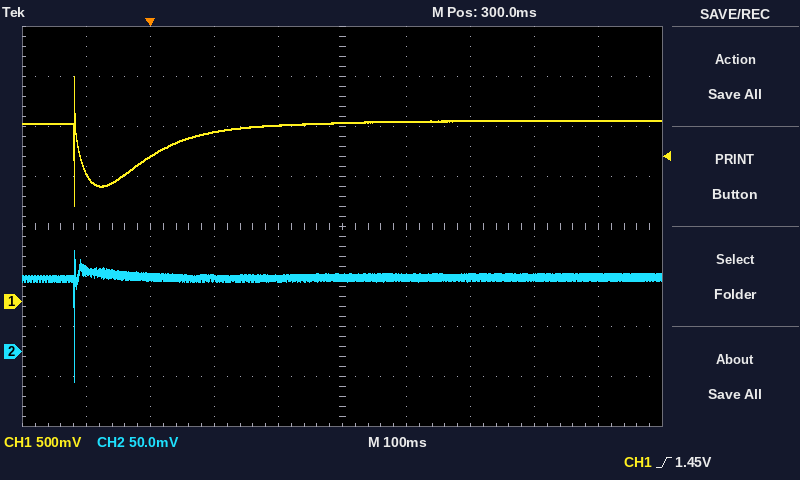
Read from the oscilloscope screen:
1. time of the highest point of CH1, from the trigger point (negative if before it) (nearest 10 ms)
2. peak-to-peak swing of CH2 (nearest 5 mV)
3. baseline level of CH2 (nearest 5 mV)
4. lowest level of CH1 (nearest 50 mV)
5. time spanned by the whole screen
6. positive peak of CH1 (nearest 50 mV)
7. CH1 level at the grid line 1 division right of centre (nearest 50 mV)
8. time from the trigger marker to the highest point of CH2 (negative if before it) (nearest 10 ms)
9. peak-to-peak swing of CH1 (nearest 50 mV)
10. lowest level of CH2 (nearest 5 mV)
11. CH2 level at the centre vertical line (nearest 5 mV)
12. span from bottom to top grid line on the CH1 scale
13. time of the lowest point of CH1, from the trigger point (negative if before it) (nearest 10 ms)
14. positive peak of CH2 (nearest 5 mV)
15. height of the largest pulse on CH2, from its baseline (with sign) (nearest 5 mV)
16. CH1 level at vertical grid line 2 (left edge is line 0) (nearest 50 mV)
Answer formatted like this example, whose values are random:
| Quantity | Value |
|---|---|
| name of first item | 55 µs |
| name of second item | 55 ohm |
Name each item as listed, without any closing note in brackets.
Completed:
| Quantity | Value |
|---|---|
| time of the highest point of CH1, from the trigger point (negative if before it) | -120 ms |
| peak-to-peak swing of CH2 | 130 mV |
| baseline level of CH2 | 75 mV |
| lowest level of CH1 | 950 mV |
| time spanned by the whole screen | 1 s |
| positive peak of CH1 | 2.25 V |
| CH1 level at the grid line 1 division right of centre | 1.80 V |
| time from the trigger marker to the highest point of CH2 (negative if before it) | -120 ms |
| peak-to-peak swing of CH1 | 1.30 V |
| lowest level of CH2 | -30 mV |
| CH2 level at the centre vertical line | 75 mV |
| span from bottom to top grid line on the CH1 scale | 4 V |
| time of the lowest point of CH1, from the trigger point (negative if before it) | -120 ms |
| positive peak of CH2 | 100 mV |
| height of the largest pulse on CH2, from its baseline (with sign) | -105 mV |
| CH1 level at vertical grid line 2 (left edge is line 0) | 1.45 V |
